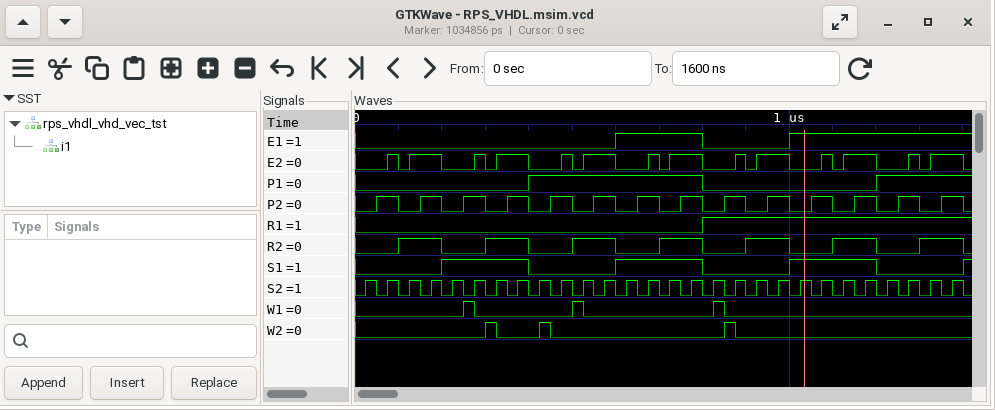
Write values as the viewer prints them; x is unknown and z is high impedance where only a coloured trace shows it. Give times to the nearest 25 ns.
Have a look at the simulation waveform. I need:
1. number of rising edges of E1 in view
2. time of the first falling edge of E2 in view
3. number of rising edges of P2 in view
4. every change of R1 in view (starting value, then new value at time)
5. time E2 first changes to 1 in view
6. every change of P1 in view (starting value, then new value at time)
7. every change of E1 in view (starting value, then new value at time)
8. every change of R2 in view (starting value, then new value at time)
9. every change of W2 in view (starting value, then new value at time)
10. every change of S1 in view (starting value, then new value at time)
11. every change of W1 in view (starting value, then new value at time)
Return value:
2
100 ns
14
0, 1 at 800 ns
75 ns
0, 1 at 400 ns, 0 at 800 ns, 1 at 1200 ns
0, 1 at 600 ns, 0 at 800 ns, 1 at 1000 ns
0, 1 at 100 ns, 0 at 200 ns, 1 at 300 ns, 0 at 400 ns, 1 at 500 ns, 0 at 600 ns, 1 at 700 ns, 0 at 800 ns, 1 at 900 ns, 0 at 1000 ns, 1 at 1100 ns, 0 at 1200 ns, 1 at 1300 ns, 0 at 1400 ns
0, 1 at 300 ns, 0 at 325 ns, 1 at 425 ns, 0 at 450 ns, 1 at 850 ns, 0 at 875 ns
0, 1 at 200 ns, 0 at 400 ns, 1 at 600 ns, 0 at 800 ns, 1 at 1000 ns, 0 at 1200 ns, 1 at 1400 ns
0, 1 at 250 ns, 0 at 275 ns, 1 at 500 ns, 0 at 525 ns, 1 at 825 ns, 0 at 850 ns
